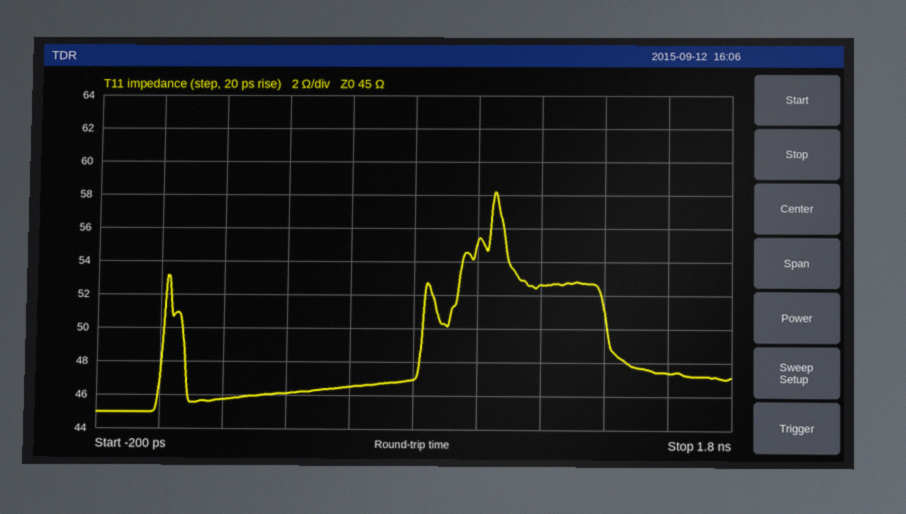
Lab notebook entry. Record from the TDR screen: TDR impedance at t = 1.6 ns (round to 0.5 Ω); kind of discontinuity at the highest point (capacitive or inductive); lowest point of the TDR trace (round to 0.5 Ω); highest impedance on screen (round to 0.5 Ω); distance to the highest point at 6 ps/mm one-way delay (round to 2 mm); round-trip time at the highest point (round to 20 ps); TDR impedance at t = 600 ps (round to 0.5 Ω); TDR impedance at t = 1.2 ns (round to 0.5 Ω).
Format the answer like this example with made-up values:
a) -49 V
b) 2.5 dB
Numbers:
a) 47.5 Ω
b) inductive
c) 45.0 Ω
d) 58.0 Ω
e) 88 mm
f) 1.06 ns
g) 46.5 Ω
h) 52.5 Ω
